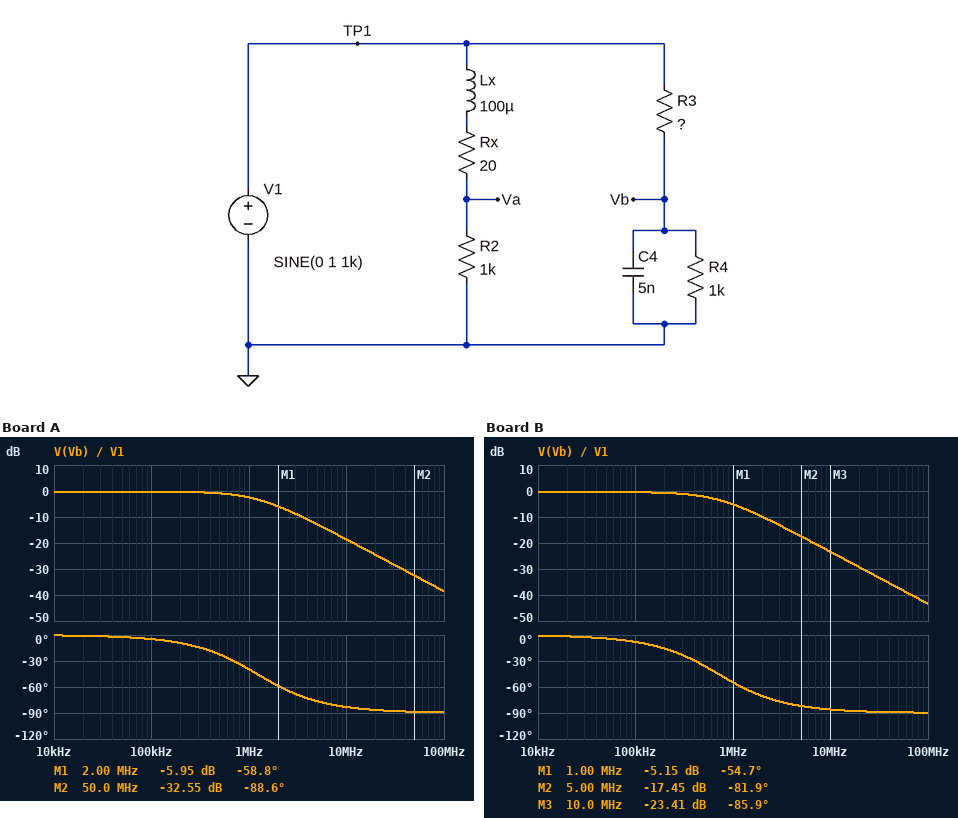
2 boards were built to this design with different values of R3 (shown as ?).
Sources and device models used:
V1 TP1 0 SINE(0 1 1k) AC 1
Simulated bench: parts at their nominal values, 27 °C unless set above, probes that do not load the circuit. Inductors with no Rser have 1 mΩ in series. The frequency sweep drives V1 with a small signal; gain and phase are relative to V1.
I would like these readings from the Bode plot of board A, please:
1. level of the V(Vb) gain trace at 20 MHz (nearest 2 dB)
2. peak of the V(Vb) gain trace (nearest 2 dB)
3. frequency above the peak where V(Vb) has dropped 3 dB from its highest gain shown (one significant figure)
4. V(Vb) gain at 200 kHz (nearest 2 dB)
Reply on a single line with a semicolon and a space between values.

-24 dB; 0 dB; 1 MHz; 0 dB
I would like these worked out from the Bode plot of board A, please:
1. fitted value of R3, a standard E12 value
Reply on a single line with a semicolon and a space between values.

27 Ω
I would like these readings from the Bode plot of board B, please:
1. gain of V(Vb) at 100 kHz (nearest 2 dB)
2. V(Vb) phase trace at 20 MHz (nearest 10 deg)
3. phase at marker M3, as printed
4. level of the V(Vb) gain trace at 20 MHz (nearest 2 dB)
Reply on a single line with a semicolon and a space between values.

0 dB; -90 deg; -85.9 deg; -30 dB
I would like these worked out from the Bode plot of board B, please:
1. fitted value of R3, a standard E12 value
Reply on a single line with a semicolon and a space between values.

47 Ω
